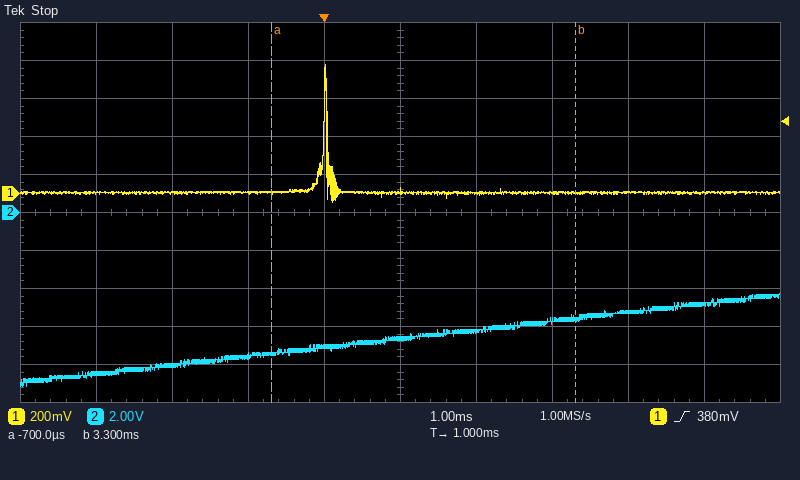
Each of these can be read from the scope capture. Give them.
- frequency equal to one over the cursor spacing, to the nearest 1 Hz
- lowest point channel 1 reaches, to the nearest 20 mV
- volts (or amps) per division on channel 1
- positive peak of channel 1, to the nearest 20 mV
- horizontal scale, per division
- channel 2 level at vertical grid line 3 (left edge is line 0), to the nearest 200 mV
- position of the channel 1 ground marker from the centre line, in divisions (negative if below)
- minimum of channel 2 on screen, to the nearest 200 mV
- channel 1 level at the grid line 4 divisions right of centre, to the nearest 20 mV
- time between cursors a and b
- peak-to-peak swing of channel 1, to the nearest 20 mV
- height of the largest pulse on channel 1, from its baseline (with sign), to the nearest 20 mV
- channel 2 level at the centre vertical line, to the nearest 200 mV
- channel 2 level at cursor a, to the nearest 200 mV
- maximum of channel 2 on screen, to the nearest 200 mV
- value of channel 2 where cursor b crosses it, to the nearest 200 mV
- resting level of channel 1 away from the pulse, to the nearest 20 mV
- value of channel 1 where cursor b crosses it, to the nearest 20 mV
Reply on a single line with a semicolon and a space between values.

250 Hz; -40 mV; 200 mV; 680 mV; 1 ms; -7.6 V; +0.5 div; -9.2 V; 0 mV; 4.0 ms; 720 mV; +680 mV; -6.6 V; -7.4 V; -4.2 V; -5.6 V; 0 mV; 0 mV
